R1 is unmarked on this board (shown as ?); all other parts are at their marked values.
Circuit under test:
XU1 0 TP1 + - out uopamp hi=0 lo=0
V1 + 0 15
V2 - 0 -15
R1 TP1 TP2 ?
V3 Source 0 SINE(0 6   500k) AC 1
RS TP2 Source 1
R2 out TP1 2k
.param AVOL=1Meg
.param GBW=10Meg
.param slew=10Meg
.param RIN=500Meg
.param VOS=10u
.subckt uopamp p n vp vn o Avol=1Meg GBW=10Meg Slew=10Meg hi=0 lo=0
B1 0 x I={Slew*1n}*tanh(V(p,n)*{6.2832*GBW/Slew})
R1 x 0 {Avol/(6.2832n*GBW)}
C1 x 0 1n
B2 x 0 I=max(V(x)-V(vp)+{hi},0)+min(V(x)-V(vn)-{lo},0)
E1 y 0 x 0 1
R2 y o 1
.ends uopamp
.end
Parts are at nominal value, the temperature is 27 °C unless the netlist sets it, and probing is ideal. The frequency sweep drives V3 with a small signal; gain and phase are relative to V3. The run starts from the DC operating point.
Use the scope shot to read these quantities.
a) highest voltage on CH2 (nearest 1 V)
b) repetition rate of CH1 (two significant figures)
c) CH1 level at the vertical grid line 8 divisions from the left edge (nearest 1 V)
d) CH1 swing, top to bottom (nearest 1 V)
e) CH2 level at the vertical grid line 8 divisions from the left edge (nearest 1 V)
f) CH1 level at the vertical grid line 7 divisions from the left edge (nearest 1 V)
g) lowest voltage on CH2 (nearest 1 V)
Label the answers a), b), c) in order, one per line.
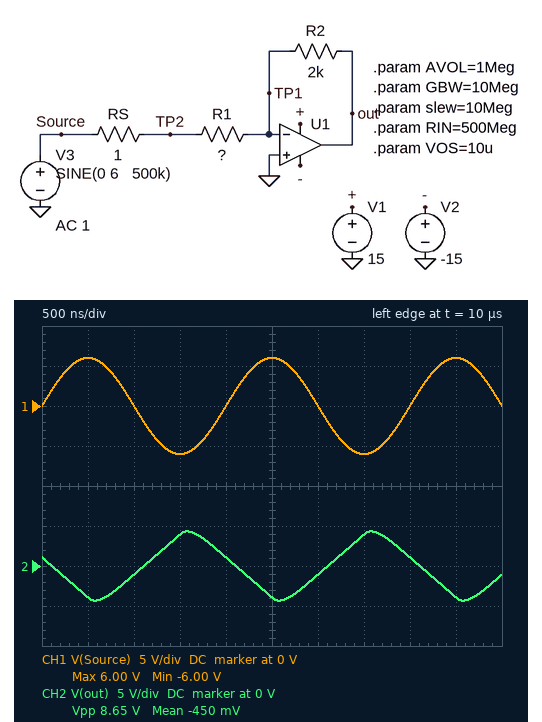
a) 4 V
b) 500 kHz
c) 0 V
d) 12 V
e) 1 V
f) -6 V
g) -4 V
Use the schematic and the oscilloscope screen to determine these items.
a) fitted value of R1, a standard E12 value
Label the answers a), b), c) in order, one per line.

a) 2.7 kΩ
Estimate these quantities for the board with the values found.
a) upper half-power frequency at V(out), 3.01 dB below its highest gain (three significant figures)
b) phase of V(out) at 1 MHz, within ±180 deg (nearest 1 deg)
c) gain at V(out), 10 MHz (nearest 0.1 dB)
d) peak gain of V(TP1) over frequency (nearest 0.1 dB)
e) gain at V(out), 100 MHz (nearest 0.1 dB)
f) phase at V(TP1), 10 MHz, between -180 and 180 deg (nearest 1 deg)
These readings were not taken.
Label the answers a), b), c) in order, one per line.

a) 5.74 MHz
b) 170 deg
c) -8.7 dB
d) -7.4 dB
e) -27.4 dB
f) 30 deg
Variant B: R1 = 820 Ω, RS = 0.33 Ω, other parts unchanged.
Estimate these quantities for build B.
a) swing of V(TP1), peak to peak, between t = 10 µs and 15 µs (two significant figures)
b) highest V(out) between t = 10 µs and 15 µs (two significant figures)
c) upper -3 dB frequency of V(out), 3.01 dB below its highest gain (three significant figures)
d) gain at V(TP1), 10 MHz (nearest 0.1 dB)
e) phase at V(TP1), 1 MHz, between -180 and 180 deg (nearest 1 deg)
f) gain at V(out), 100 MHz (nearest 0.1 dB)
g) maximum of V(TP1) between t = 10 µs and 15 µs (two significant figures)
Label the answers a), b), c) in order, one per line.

a) 8.1 V
b) 4.9 V
c) 2.91 MHz
d) -3.3 dB
e) 71 deg
f) -23.0 dB
g) 4.0 V
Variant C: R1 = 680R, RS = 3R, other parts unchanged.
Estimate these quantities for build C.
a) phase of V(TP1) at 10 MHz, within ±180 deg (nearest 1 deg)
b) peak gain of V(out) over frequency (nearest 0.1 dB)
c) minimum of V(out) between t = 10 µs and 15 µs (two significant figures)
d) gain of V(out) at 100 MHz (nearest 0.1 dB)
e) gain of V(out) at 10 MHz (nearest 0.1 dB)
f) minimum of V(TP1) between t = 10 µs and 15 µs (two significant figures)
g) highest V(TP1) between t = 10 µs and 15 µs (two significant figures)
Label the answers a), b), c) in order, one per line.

a) 14 deg
b) 9.3 dB
c) -5.0 V
d) -22.6 dB
e) -2.8 dB
f) -4.3 V
g) 4.3 V
